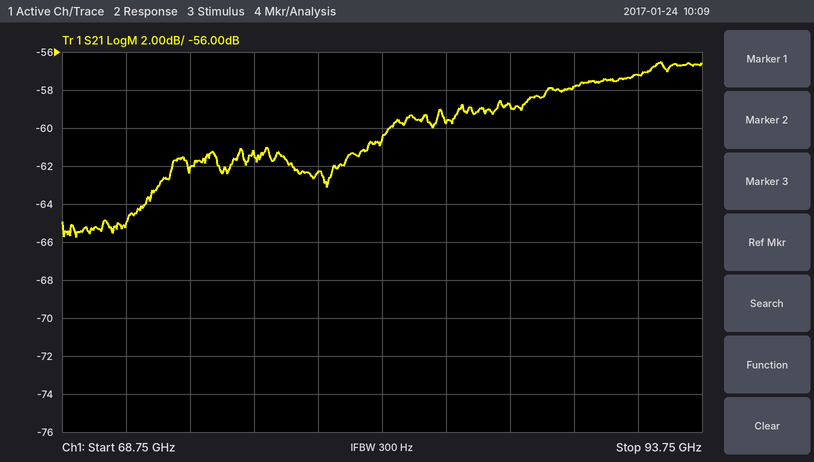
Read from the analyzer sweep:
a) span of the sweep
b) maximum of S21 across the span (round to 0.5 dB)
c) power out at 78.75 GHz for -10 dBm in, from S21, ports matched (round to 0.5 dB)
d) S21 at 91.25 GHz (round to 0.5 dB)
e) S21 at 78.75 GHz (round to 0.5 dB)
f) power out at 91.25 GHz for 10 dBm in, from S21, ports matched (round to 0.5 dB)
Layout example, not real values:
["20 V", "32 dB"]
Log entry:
["25 GHz", "-56.5 dB", "-72.5 dBm", "-57.0 dB", "-62.5 dB", "-47.0 dBm"]
